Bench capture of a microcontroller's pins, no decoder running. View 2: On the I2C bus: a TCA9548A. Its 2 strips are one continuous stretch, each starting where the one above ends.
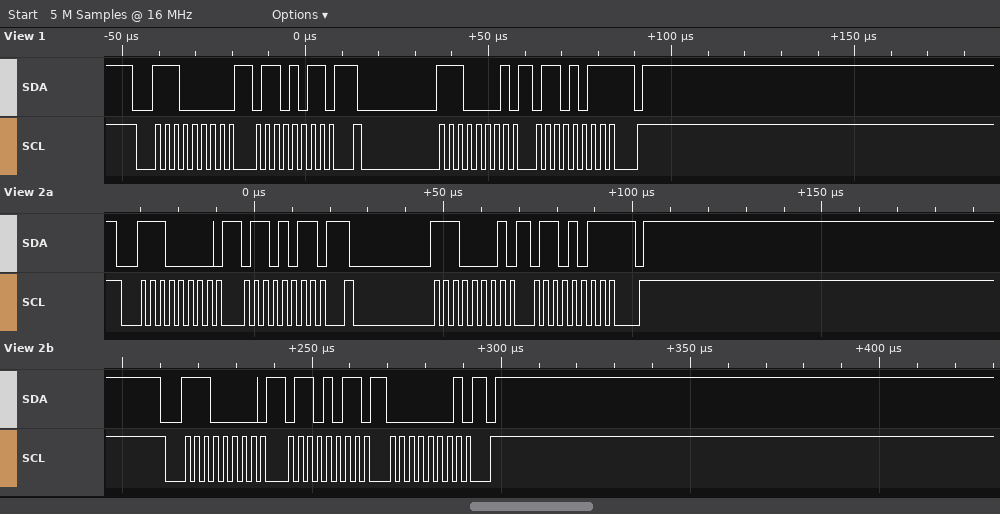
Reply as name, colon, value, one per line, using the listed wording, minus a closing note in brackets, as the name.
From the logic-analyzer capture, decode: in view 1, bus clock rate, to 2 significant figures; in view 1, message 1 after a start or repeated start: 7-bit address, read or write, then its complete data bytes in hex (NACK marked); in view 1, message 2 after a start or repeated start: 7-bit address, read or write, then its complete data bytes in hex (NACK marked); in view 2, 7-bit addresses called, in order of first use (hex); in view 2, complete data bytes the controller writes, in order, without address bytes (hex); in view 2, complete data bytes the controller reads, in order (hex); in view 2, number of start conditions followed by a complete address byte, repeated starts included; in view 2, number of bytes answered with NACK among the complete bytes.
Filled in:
in view 1, bus clock rate, to 2 significant figures: 400 kHz
in view 1, message 1 after a start or repeated start: 7-bit address, read or write, then its complete data bytes in hex: 0x70 write: 6B
in view 1, message 2 after a start or repeated start: 7-bit address, read or write, then its complete data bytes in hex: 0x70 read: 6B NACK
in view 2, 7-bit addresses called, in order of first use: 0x70
in view 2, complete data bytes the controller writes, in order, without address bytes: 6B 6B 01
in view 2, complete data bytes the controller reads, in order: 6B
in view 2, number of start conditions followed by a complete address byte, repeated starts included: 3
in view 2, number of bytes answered with NACK among the complete bytes: 1
